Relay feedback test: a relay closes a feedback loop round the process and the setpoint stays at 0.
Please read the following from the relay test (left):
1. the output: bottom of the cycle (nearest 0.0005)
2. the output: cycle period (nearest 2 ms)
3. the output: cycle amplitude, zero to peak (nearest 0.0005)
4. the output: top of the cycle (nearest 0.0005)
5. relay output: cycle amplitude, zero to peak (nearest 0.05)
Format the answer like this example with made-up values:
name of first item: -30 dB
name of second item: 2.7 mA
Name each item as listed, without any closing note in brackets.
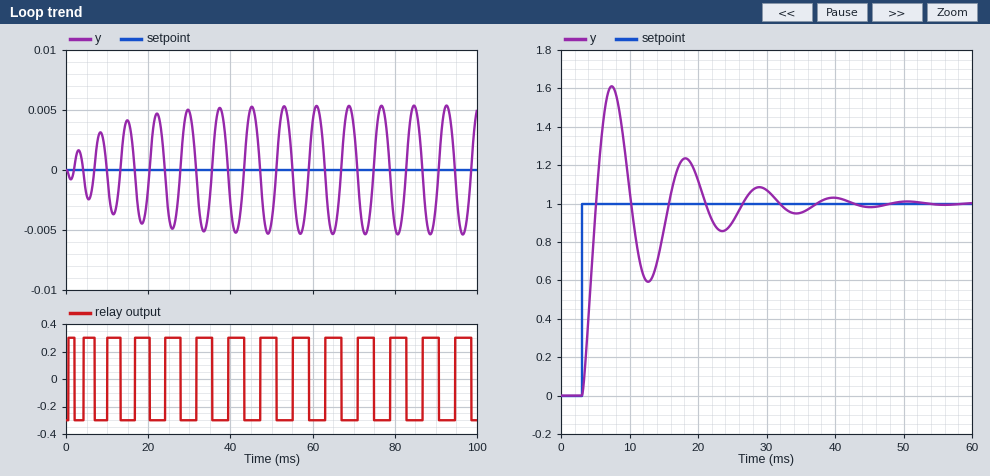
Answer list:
the output: bottom of the cycle: -0.0055
the output: cycle period: 8 ms
the output: cycle amplitude, zero to peak: 0.0055
the output: top of the cycle: 0.0055
relay output: cycle amplitude, zero to peak: 0.30
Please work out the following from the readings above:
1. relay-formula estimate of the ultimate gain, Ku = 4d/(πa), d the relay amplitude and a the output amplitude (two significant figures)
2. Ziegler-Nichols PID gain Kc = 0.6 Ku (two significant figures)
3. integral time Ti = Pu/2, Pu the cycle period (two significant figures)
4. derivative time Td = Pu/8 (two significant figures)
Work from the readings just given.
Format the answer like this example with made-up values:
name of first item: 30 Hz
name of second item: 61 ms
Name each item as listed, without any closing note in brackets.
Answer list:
relay-formula estimate of the ultimate gain, Ku = 4d/(πa), d the relay amplitude and a the output amplitude: 69
Ziegler-Nichols PID gain Kc = 0.6 Ku: 41
integral time Ti = Pu/2, Pu the cycle period: 4.0 ms
derivative time Td = Pu/8: 1.0 ms
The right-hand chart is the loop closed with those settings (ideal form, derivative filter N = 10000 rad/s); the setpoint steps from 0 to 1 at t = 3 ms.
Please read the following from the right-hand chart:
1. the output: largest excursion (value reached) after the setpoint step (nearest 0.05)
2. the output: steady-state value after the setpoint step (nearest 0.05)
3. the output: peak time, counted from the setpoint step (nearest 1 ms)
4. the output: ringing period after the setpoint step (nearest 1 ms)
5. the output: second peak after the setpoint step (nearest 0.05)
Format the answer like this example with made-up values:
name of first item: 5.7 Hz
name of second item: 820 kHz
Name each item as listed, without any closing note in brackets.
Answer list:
the output: largest excursion (value reached) after the setpoint step: 1.60
the output: steady-state value after the setpoint step: 1.00
the output: peak time, counted from the setpoint step: 4 ms
the output: ringing period after the setpoint step: 11 ms
the output: second peak after the setpoint step: 1.25
